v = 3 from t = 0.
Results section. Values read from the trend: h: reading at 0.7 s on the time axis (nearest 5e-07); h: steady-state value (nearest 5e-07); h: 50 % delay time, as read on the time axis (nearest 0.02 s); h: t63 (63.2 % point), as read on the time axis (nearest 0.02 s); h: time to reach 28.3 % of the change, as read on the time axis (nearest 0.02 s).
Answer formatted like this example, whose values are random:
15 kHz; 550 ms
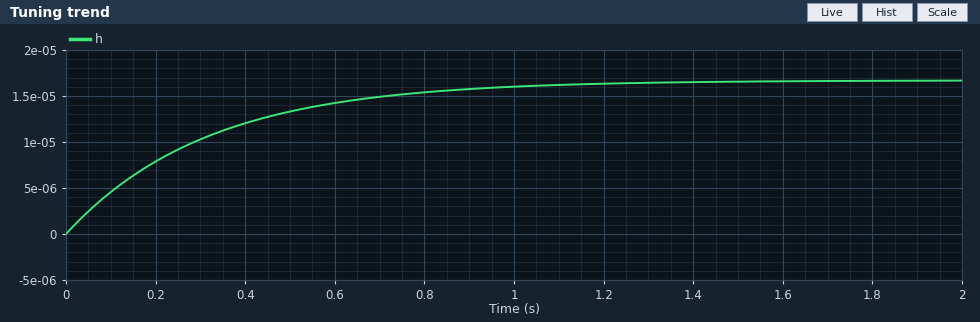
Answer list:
0.0000150; 0.0000165; 0.22 s; 0.32 s; 0.10 s
